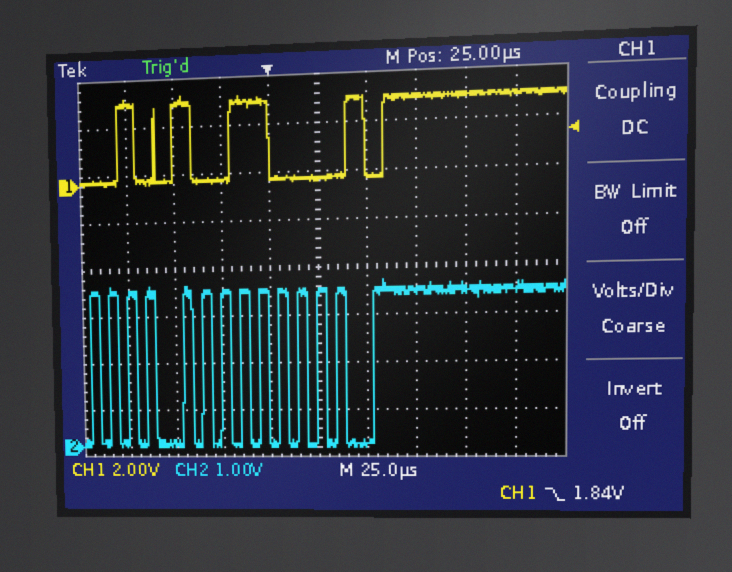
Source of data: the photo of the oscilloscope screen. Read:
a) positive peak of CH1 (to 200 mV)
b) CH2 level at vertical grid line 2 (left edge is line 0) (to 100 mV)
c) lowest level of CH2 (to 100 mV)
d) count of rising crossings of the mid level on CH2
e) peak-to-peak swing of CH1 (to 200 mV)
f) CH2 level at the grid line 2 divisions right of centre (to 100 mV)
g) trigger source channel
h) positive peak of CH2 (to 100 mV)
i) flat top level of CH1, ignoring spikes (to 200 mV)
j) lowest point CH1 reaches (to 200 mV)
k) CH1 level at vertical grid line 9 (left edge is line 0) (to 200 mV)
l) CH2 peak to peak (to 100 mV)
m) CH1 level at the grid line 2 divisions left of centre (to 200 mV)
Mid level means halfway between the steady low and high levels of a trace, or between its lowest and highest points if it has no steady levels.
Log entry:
3.6 V
100 mV
0.0 V
14
3.6 V
3.3 V
CH1
3.5 V
3.4 V
0.0 V
3.4 V
3.5 V
200 mV
